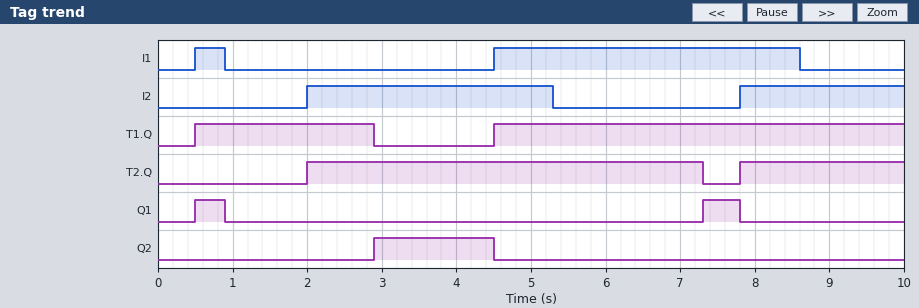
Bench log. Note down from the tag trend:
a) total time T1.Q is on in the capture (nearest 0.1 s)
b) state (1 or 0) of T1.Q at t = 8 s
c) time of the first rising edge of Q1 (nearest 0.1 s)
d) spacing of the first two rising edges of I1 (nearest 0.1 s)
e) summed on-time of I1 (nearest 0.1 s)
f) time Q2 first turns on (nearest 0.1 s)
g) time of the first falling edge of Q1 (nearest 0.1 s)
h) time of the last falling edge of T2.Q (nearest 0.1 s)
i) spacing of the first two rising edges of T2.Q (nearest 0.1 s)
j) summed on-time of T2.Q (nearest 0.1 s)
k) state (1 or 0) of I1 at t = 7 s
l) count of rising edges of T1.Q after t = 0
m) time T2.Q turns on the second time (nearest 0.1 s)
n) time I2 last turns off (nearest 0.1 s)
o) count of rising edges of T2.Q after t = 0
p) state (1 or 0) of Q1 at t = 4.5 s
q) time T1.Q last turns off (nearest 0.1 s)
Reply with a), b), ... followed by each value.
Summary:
a) 7.9 s
b) 1
c) 0.5 s
d) 4.0 s
e) 4.5 s
f) 2.9 s
g) 0.9 s
h) 7.3 s
i) 5.8 s
j) 7.5 s
k) 1
l) 2
m) 7.8 s
n) 5.3 s
o) 2
p) 0
q) 2.9 s
